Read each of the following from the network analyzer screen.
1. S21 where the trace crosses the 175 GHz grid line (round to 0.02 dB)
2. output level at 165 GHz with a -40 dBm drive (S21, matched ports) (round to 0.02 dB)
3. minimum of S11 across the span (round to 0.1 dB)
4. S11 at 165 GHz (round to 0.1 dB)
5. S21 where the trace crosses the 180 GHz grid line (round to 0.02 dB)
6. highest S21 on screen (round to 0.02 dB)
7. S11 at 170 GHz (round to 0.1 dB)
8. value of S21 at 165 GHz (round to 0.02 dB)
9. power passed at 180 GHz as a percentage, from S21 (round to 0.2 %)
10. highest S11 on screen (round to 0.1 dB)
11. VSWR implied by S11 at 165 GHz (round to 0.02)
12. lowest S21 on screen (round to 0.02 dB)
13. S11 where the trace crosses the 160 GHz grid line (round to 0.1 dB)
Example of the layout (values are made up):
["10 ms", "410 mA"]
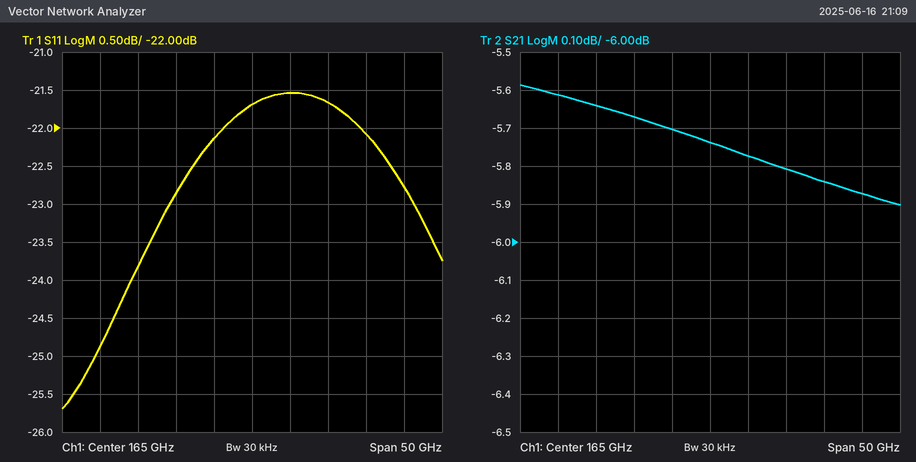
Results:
["-5.80 dB", "-45.74 dBm", "-25.7 dB", "-21.7 dB", "-5.84 dB", "-5.58 dB", "-21.5 dB", "-5.74 dB", "26.0 %", "-21.5 dB", "1.18", "-5.90 dB", "-22.1 dB"]
